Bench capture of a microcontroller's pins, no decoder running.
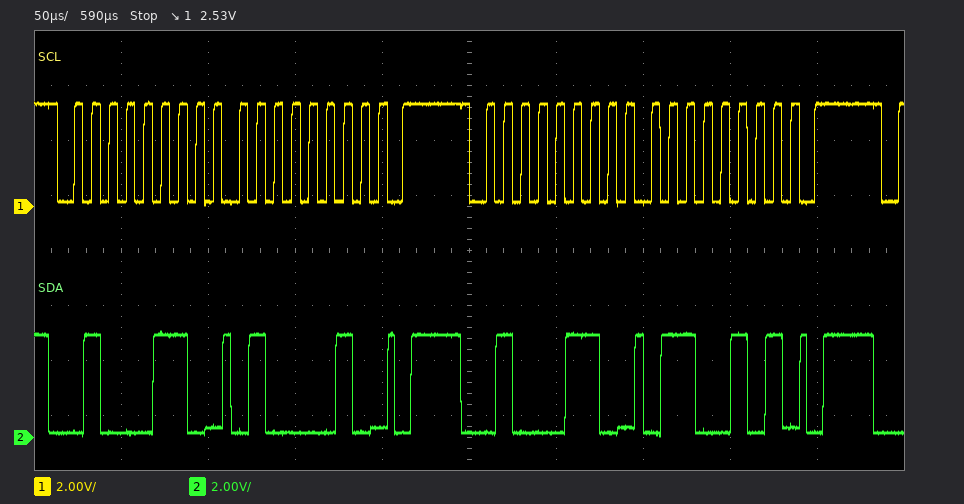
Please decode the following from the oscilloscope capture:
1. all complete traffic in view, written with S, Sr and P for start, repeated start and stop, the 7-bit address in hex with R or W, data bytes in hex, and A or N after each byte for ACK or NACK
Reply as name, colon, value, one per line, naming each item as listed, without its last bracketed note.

all complete traffic in view, written with S, Sr and P for start, repeated start and stop, the 7-bit address in hex with R or W, data bytes in hex, and A or N after each byte for ACK or NACK: S 23W A 42 A P S 23W A 65 A P
